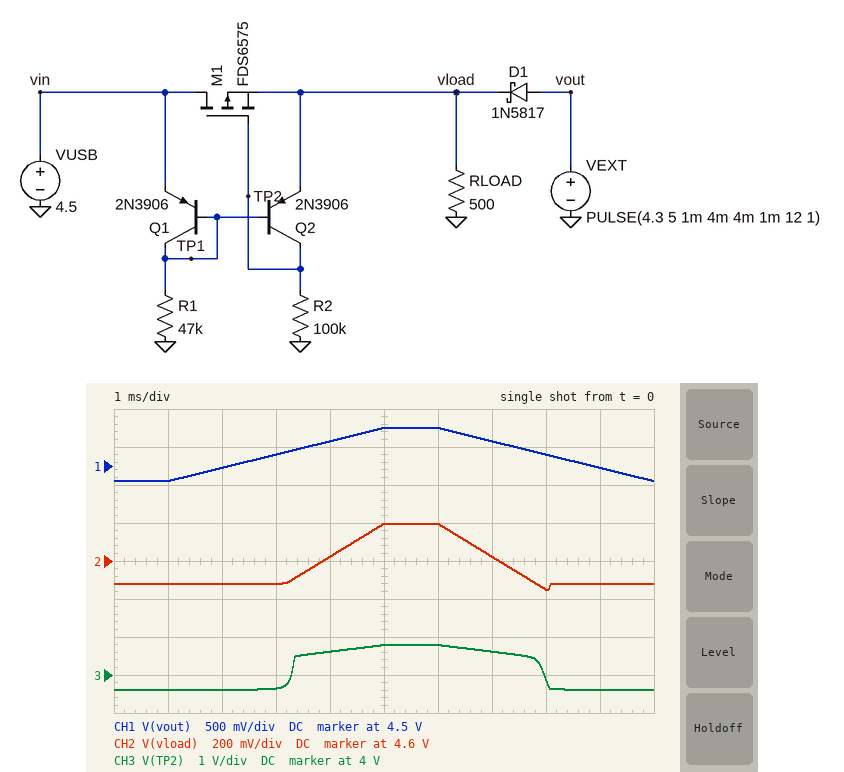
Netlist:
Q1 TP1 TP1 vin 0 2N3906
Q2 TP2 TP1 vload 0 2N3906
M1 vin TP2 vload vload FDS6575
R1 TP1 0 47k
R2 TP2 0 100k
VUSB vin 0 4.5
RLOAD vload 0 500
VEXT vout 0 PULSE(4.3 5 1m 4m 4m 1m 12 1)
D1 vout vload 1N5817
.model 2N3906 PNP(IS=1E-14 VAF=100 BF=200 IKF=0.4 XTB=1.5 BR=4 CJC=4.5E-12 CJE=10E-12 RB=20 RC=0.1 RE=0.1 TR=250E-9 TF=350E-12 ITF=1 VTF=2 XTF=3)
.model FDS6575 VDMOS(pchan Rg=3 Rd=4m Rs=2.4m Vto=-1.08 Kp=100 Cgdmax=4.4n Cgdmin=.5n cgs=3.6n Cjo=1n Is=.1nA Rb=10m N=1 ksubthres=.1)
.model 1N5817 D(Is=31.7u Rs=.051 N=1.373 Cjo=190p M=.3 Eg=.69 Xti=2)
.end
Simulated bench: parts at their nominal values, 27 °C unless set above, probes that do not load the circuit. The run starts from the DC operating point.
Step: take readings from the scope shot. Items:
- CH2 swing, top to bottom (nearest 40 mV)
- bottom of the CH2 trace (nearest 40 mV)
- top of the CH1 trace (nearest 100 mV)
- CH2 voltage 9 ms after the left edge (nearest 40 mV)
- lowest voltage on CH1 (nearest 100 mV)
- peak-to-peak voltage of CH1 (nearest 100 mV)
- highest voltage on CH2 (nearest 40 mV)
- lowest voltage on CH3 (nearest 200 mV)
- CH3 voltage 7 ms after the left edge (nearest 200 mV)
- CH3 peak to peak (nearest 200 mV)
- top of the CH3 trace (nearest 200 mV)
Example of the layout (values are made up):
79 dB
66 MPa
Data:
360 mV
4.44 V
5.0 V
4.48 V
4.3 V
700 mV
4.80 V
3.6 V
4.6 V
1.2 V
4.8 V
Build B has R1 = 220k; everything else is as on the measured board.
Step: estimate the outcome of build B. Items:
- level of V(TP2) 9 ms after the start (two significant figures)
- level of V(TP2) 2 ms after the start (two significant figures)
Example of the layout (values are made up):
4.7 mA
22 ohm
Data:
2.2 V
1.8 V
